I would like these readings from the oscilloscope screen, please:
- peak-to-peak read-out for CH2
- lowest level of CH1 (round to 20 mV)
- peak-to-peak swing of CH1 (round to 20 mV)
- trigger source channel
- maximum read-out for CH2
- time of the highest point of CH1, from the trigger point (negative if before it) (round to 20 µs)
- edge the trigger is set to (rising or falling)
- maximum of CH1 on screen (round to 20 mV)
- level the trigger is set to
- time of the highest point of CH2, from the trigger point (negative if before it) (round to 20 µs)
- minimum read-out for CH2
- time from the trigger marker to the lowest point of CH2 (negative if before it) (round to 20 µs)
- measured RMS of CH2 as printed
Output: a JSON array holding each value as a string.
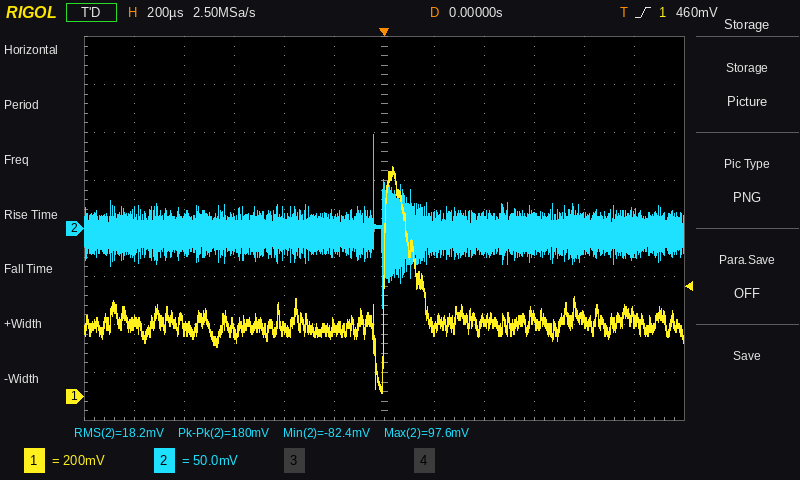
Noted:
["180 mV", "20 mV", "940 mV", "CH1", "97.6 mV", "+40 µs", "rising", "960 mV", "460 mV", "-40 µs", "-82.4 mV", "0 µs", "18.2 mV"]
